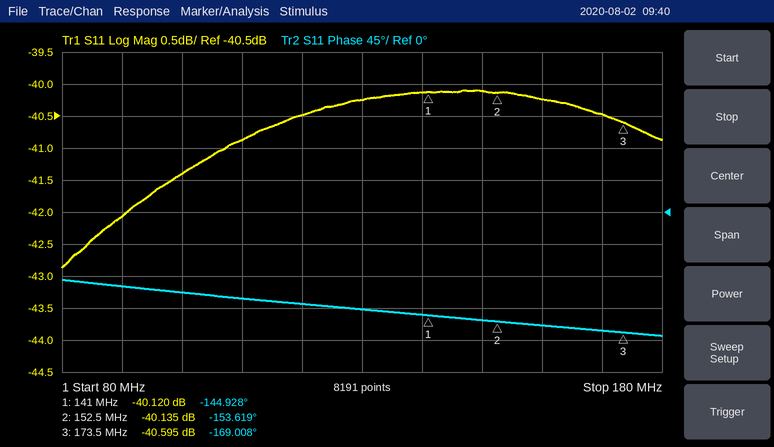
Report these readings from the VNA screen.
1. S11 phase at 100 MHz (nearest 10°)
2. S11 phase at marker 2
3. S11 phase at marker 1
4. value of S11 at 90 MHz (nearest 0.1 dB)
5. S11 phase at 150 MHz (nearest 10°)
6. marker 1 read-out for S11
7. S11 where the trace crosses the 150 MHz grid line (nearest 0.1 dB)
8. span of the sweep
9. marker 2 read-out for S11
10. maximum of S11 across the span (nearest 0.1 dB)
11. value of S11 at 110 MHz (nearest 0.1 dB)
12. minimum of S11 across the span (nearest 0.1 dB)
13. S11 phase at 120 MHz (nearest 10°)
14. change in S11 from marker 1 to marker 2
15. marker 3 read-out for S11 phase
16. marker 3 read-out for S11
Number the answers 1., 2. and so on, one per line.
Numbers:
1. -110°
2. -153.619°
3. -144.928°
4. -42.1 dB
5. -150°
6. -40.120 dB
7. -40.1 dB
8. 100 MHz
9. -40.135 dB
10. -40.1 dB
11. -40.9 dB
12. -42.9 dB
13. -130°
14. -0.015 dB
15. -169.008°
16. -40.595 dB
